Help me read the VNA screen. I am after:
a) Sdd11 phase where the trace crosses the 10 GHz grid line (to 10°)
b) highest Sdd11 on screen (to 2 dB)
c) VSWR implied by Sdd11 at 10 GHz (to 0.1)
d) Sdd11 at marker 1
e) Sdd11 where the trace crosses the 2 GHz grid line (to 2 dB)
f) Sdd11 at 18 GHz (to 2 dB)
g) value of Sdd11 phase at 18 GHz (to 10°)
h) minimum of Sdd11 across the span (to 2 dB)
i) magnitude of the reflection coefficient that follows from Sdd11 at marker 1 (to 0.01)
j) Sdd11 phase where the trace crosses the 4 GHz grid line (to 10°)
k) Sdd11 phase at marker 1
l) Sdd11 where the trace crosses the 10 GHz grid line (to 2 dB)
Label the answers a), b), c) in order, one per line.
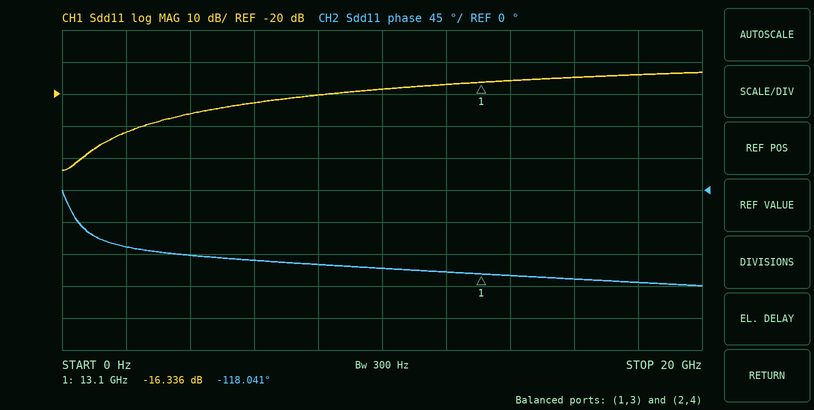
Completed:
a) -110°
b) -14 dB
c) 1.3
d) -16.336 dB
e) -32 dB
f) -14 dB
g) -130°
h) -44 dB
i) 0.15
j) -90°
k) -118.041°
l) -18 dB
